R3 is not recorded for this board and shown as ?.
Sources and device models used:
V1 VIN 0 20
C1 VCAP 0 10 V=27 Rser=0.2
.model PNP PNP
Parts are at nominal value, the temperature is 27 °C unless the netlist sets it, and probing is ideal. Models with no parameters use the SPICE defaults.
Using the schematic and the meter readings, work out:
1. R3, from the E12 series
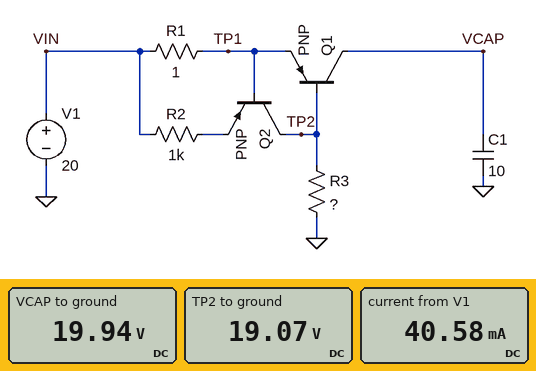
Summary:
470 Ω
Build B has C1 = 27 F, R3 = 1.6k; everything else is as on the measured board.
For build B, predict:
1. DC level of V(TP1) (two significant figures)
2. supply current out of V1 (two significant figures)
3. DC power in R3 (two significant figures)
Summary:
20 V
12 mA
230 mW
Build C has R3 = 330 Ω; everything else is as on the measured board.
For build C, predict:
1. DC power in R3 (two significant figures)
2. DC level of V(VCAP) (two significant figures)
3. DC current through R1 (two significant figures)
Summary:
1.1 W
20 V
58 mA
